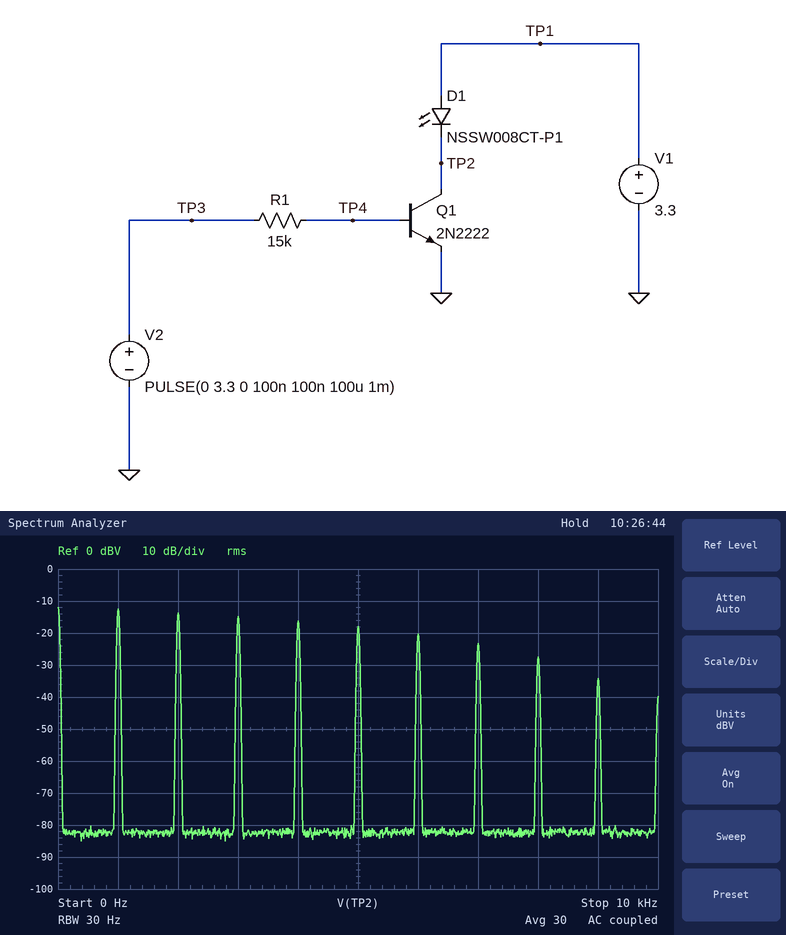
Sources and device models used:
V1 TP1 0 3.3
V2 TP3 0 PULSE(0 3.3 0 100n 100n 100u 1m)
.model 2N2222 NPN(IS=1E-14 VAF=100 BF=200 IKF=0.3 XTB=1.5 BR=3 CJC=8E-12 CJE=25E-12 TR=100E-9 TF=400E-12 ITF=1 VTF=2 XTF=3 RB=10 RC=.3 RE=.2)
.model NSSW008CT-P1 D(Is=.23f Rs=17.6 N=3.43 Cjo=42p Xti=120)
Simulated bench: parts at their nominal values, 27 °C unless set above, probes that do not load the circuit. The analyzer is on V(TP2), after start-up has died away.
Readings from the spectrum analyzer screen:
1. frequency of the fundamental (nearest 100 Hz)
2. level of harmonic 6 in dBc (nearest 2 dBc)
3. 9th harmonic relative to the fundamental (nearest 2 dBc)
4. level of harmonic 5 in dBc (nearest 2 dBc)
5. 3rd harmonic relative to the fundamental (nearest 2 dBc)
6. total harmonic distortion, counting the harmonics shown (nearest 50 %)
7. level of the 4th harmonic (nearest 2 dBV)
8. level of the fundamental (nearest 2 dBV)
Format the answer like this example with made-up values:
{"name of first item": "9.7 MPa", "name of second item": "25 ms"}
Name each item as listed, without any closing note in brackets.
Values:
{"frequency of the fundamental": "1.0 kHz", "level of harmonic 6 in dBc": "-8 dBc", "9th harmonic relative to the fundamental": "-22 dBc", "level of harmonic 5 in dBc": "-6 dBc", "3rd harmonic relative to the fundamental": "-2 dBc", "total harmonic distortion, counting the harmonics shown": "150 %", "level of the 4th harmonic": "-16 dBV", "level of the fundamental": "-12 dBV"}
